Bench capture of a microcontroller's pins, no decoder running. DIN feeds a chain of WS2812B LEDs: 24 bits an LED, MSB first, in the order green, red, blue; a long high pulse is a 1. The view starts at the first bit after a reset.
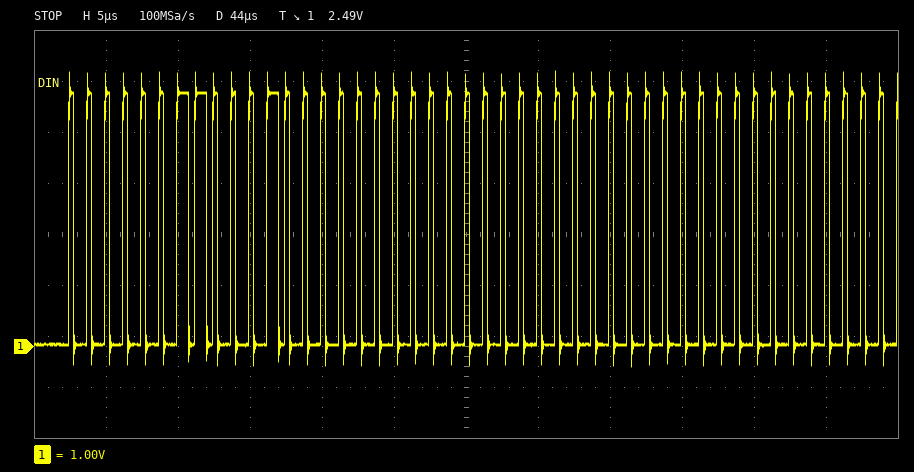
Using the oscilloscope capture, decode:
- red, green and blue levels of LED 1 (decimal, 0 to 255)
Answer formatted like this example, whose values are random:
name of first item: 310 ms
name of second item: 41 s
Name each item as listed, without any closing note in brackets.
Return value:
red, green and blue levels of LED 1: 16, 3, 0
